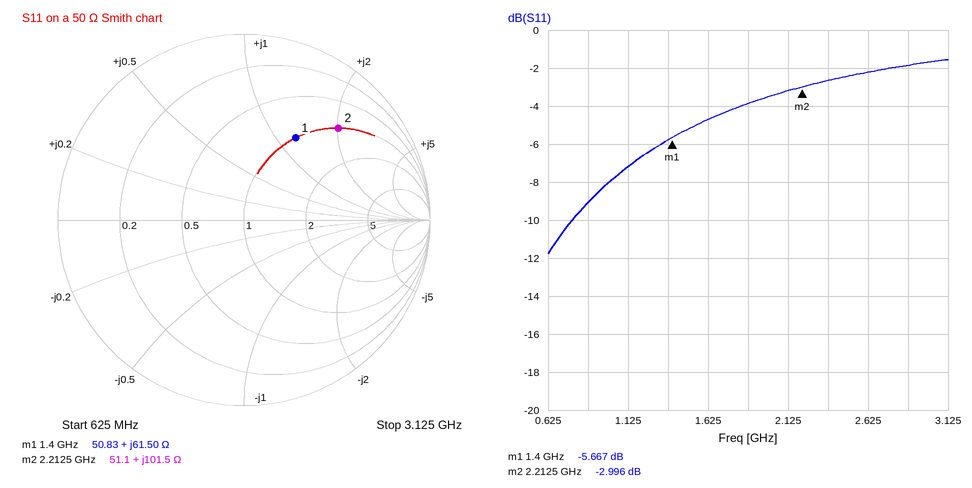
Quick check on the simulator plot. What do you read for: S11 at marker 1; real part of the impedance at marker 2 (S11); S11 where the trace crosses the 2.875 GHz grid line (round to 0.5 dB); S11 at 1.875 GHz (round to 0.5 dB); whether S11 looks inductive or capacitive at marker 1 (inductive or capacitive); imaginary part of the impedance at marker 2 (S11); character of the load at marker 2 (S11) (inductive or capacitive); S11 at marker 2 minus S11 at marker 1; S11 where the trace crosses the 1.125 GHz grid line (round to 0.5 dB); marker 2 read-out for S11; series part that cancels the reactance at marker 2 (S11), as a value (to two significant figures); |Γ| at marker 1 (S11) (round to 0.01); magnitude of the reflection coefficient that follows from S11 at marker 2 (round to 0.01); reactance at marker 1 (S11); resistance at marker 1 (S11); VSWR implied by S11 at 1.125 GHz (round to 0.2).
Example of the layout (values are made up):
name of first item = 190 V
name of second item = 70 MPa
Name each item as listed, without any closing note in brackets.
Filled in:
S11 at marker 1 = -5.667 dB
real part of the impedance at marker 2 = 51.1 Ω
S11 where the trace crosses the 2.875 GHz grid line = -2.0 dB
S11 at 1.875 GHz = -4.0 dB
whether S11 looks inductive or capacitive at marker 1 = inductive
imaginary part of the impedance at marker 2 = +101.5 Ω
character of the load at marker 2 (S11) = inductive
S11 at marker 2 minus S11 at marker 1 = 2.671 dB
S11 where the trace crosses the 1.125 GHz grid line = -7.0 dB
marker 2 read-out for S11 = -2.996 dB
series part that cancels the reactance at marker 2 (S11), as a value = 710 fF
|Γ| at marker 1 (S11) = 0.52
magnitude of the reflection coefficient that follows from S11 at marker 2 = 0.71
reactance at marker 1 = +61.50 Ω
resistance at marker 1 = 50.83 Ω
VSWR implied by S11 at 1.125 GHz = 2.6
